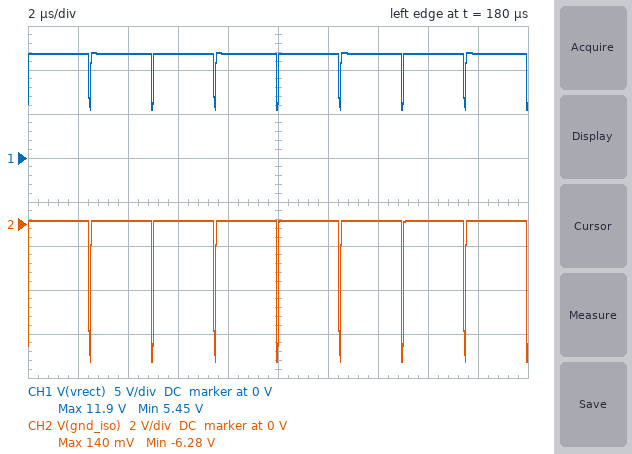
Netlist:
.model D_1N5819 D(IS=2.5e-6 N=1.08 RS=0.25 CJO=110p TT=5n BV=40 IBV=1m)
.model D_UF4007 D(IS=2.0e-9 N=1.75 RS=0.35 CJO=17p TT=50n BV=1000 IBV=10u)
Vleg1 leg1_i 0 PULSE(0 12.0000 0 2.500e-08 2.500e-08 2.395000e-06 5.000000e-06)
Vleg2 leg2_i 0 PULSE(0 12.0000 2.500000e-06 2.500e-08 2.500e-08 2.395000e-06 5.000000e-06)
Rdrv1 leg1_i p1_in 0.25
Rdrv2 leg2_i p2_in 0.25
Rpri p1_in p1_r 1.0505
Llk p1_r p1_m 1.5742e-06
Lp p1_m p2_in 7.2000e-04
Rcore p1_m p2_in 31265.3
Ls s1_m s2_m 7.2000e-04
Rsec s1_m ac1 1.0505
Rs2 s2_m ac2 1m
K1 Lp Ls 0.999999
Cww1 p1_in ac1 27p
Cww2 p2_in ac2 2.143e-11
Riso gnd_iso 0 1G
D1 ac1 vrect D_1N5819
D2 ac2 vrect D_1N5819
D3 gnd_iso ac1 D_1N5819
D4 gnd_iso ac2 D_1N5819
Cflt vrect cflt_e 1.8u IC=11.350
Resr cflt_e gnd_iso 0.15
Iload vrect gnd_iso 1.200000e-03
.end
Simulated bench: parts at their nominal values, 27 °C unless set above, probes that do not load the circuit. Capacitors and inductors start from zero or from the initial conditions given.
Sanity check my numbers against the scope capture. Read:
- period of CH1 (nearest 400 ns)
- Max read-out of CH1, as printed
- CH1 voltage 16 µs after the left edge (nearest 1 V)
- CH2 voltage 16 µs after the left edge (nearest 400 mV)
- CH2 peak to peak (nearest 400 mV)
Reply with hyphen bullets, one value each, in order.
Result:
- 2.4 µs
- 11.9 V
- 12 V
- 0 V
- 6.4 V
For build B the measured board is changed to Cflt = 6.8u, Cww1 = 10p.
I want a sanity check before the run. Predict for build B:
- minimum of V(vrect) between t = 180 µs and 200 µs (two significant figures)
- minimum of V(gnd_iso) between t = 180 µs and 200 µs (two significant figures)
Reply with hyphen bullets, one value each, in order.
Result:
- 4.3 V
- -7.3 V
